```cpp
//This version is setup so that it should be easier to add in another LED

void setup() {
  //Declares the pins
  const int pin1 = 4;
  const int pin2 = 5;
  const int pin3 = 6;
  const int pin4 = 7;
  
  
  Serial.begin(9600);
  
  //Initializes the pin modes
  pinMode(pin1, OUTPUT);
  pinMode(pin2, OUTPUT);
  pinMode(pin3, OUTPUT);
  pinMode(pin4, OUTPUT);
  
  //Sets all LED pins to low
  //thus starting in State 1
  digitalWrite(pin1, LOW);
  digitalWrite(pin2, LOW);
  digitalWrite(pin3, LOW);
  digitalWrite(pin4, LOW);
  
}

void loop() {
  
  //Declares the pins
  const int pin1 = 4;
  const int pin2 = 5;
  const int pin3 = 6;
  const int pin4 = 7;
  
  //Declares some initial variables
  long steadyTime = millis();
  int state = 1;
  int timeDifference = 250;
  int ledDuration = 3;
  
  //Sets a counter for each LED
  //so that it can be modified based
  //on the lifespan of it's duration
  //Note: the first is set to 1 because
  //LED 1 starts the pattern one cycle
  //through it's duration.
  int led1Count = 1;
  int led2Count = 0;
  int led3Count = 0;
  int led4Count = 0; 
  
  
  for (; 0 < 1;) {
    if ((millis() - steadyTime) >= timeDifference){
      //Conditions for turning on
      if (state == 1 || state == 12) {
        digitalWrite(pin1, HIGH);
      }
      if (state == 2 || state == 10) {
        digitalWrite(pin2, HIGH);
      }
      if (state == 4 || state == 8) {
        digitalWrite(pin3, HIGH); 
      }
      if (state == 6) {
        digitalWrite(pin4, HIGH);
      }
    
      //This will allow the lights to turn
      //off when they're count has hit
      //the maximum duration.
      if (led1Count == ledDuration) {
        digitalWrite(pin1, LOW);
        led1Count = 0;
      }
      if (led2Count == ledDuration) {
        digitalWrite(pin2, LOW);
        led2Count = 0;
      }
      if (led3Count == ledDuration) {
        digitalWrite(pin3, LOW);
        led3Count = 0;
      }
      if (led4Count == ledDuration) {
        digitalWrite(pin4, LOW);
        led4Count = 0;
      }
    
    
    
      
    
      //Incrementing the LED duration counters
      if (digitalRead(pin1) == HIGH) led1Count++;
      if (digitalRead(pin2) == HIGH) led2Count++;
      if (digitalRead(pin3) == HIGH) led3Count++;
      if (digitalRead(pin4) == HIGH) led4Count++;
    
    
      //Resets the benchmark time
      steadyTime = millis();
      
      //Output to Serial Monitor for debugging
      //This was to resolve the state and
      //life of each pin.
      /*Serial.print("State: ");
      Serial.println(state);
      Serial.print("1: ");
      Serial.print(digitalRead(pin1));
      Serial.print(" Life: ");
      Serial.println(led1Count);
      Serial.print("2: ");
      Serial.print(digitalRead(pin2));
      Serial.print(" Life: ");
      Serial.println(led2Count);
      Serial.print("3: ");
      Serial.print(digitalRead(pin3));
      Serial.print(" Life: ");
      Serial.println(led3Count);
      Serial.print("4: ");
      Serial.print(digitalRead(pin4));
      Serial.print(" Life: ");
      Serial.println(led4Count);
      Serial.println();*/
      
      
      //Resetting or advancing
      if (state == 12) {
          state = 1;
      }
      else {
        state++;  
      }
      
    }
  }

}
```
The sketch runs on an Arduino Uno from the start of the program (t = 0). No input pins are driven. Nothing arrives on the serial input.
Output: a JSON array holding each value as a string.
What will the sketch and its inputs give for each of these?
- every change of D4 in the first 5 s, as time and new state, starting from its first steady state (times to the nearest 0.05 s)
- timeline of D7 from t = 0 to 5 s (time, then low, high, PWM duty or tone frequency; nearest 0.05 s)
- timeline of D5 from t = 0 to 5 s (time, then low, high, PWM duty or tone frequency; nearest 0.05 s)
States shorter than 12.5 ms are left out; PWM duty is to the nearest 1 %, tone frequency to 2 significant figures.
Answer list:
["0 s low; 0.25 s high; 0.75 s low; 3 s high; 3.75 s low", "0 s low; 1.5 s high; 2.25 s low; 4.5 s high", "0 s low; 0.5 s high; 1.25 s low; 2.5 s high; 3.25 s low; 3.5 s high; 4.25 s low"]
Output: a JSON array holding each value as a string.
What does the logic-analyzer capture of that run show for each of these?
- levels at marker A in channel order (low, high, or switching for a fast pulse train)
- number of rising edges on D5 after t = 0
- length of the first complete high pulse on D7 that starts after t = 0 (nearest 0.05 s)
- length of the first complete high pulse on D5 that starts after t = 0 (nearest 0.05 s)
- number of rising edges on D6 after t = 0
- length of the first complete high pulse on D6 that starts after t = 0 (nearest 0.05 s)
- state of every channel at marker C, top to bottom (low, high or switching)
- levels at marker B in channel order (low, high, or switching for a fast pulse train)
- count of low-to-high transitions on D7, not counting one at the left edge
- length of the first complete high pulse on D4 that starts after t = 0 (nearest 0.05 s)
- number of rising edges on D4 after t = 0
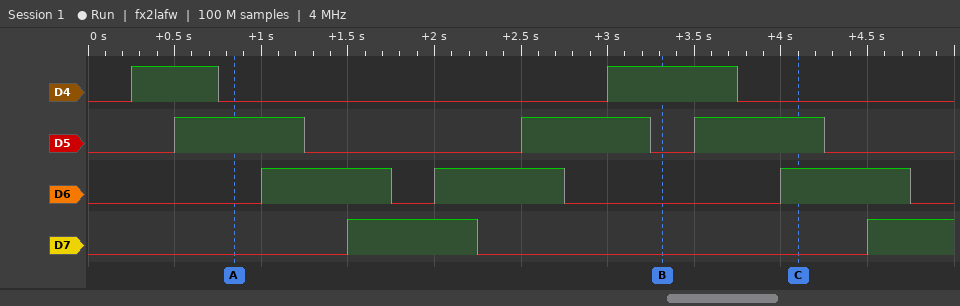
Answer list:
["D4 low, D5 high, D6 low, D7 low", "3", "0.75 s", "0.75 s", "3", "0.75 s", "D4 low, D5 high, D6 high, D7 low", "D4 high, D5 low, D6 low, D7 low", "2", "0.50 s", "2"]
